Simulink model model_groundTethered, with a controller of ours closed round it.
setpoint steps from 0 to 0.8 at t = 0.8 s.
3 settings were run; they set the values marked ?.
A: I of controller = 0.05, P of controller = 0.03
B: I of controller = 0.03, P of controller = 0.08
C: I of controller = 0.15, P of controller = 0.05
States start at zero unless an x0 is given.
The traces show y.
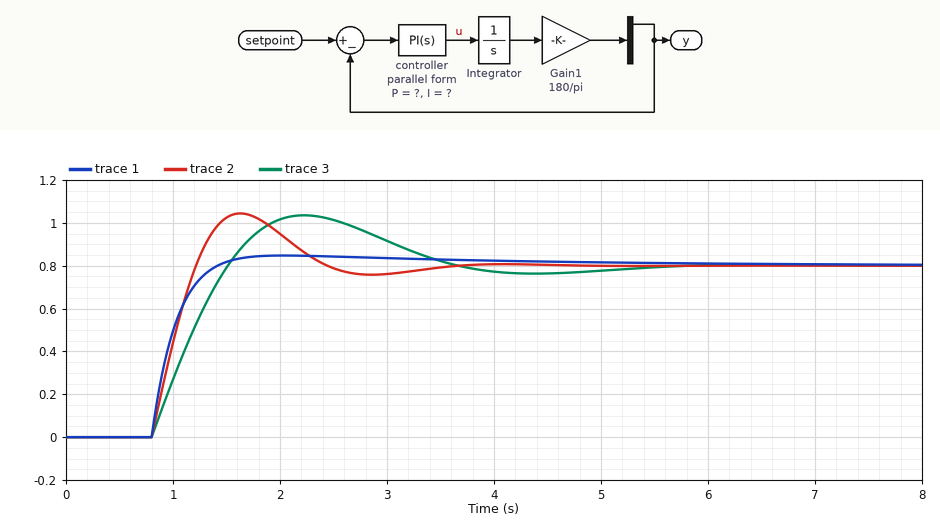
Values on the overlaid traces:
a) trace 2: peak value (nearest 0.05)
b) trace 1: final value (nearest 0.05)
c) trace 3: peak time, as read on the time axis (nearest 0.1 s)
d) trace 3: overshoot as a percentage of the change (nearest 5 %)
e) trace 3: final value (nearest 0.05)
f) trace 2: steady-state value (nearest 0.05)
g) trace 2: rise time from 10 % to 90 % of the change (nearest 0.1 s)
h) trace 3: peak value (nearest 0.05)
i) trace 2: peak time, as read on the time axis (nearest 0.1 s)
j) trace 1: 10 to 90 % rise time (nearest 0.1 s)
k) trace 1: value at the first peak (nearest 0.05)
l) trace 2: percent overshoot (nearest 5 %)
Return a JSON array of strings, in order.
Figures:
["1.05", "0.80", "2.2 s", "30 %", "0.80", "0.80", "0.3 s", "1.05", "1.6 s", "0.4 s", "0.85", "30 %"]
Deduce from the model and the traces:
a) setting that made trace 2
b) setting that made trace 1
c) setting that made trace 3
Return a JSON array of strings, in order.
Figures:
["C", "B", "A"]
